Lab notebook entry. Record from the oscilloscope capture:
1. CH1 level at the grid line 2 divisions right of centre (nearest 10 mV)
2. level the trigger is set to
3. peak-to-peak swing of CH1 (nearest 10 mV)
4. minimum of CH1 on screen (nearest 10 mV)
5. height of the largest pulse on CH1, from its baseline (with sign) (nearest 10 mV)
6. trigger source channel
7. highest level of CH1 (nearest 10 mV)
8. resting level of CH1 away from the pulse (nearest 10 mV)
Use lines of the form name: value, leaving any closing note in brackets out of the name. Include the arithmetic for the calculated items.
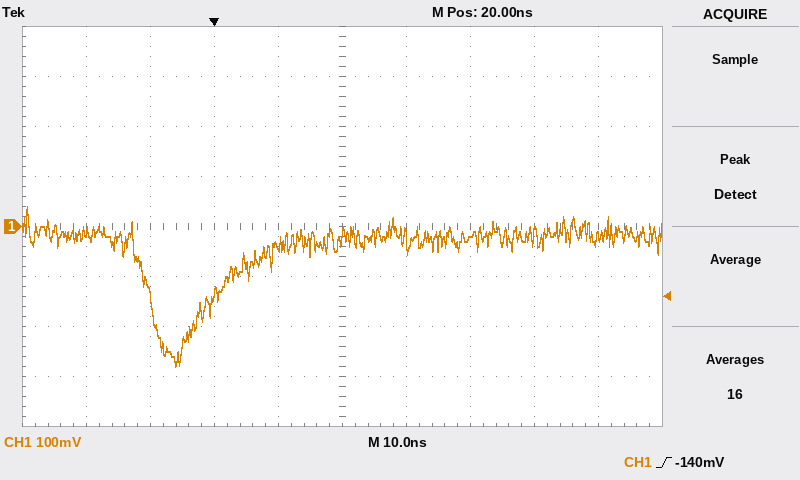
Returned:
CH1 level at the grid line 2 divisions right of centre: -20 mV
level the trigger is set to: -140 mV
peak-to-peak swing of CH1: 40 mV − (-280 mV) = 320 mV
minimum of CH1 on screen: -280 mV
height of the largest pulse on CH1, from its baseline (with sign): -280 mV − (-20 mV) = -260 mV
trigger source channel: CH1
highest level of CH1: 40 mV
resting level of CH1 away from the pulse: -20 mV
